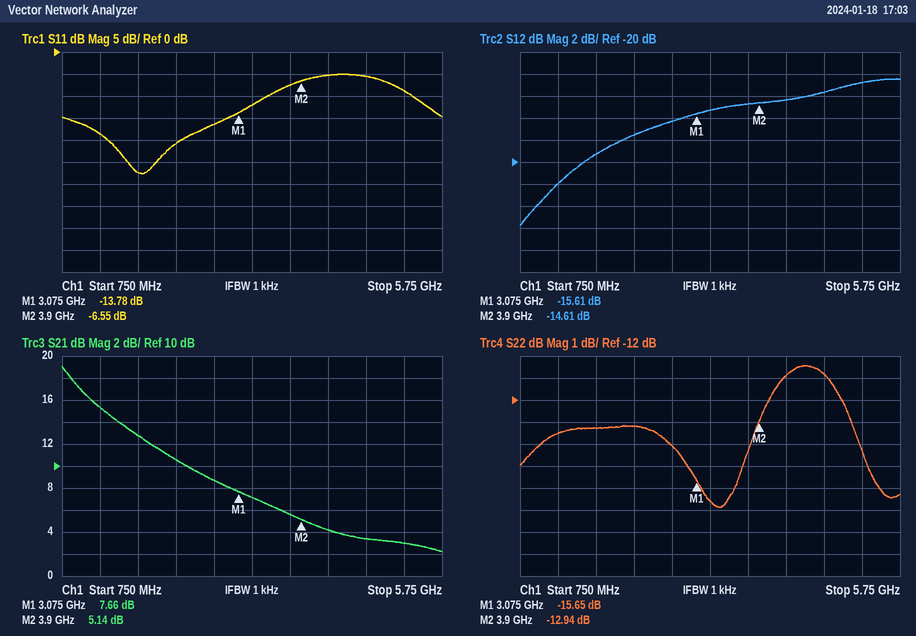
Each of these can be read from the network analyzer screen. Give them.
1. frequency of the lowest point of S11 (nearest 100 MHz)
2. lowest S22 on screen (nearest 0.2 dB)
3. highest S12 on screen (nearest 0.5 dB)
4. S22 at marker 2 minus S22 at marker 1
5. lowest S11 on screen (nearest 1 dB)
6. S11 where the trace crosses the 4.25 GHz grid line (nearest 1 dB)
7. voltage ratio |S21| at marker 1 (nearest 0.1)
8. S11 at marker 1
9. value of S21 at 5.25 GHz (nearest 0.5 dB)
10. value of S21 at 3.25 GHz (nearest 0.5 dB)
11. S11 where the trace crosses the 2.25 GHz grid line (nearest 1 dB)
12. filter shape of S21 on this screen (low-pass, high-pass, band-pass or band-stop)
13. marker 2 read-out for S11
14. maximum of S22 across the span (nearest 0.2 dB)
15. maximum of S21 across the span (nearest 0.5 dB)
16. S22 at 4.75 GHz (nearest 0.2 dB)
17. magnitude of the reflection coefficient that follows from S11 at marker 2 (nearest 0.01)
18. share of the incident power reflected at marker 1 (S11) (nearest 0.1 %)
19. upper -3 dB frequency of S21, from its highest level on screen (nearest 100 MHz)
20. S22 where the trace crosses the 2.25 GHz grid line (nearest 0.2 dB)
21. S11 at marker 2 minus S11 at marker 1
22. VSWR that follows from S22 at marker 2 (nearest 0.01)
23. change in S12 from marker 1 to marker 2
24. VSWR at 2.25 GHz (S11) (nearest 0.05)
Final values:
1.8 GHz
-16.8 dB
-12.5 dB
2.71 dB
-28 dB
-5 dB
2.4
-13.78 dB
3.0 dB
7.0 dB
-21 dB
low-pass
-6.55 dB
-10.4 dB
19.0 dB
-10.8 dB
0.47
4.2 %
1.1 GHz
-13.2 dB
7.23 dB
1.58
1.00 dB
1.20
